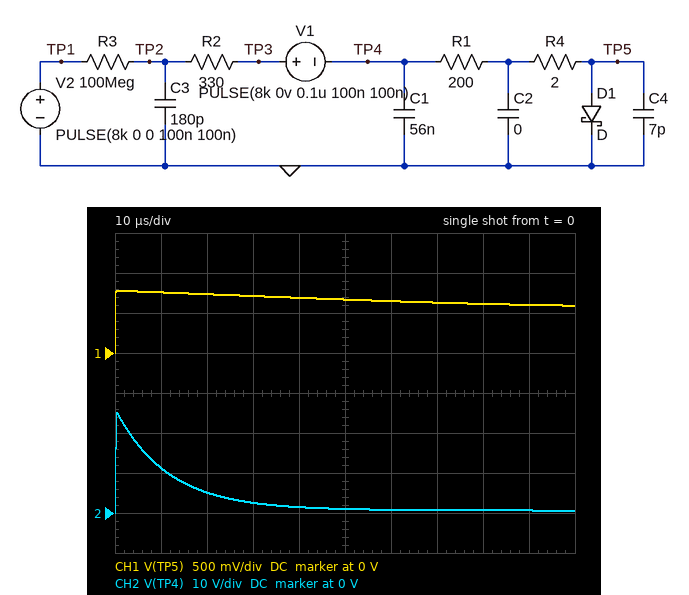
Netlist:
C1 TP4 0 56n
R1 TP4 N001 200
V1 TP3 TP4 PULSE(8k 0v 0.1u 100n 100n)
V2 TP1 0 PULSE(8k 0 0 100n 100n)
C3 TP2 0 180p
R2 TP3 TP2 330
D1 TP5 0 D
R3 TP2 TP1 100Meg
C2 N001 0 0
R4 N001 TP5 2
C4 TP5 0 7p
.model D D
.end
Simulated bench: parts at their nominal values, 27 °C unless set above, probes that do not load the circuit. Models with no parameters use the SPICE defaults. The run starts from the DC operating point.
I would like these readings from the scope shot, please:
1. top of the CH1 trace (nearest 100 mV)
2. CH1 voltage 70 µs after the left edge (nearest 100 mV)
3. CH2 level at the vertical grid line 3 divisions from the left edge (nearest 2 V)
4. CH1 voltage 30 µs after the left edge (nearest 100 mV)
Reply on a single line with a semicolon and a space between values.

800 mV; 600 mV; 2 V; 700 mV
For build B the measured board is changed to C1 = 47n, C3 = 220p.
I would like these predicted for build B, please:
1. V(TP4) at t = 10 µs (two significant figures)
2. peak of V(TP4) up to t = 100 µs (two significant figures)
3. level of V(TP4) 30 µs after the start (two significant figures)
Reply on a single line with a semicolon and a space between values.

14 V; 36 V; 2.3 V
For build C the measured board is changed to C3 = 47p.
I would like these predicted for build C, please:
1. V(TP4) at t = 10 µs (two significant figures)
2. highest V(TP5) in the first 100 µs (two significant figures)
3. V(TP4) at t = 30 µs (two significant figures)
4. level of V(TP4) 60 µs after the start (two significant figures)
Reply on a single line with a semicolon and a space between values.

3.2 V; 740 mV; 1.1 V; 670 mV
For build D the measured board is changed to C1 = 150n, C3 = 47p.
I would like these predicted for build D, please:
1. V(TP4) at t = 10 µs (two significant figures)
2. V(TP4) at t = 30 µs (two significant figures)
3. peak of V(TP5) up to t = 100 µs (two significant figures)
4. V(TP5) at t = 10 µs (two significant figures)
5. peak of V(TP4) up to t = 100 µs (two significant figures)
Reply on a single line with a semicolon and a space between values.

2.0 V; 1.4 V; 710 mV; 700 mV; 2.5 V
